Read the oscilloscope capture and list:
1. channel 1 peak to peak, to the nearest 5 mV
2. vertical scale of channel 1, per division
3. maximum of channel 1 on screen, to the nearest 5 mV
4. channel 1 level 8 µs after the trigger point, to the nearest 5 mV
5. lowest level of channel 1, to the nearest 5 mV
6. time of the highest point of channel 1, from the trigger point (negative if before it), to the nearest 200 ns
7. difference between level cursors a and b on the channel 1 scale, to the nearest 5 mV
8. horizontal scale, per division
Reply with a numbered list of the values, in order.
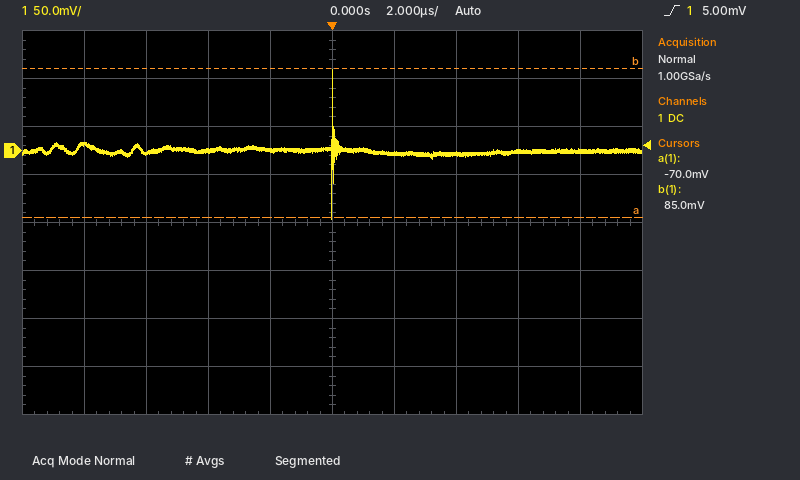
1. 155 mV
2. 50 mV
3. 85 mV
4. 0 mV
5. -70 mV
6. 0.0 µs
7. 155 mV
8. 2 µs
